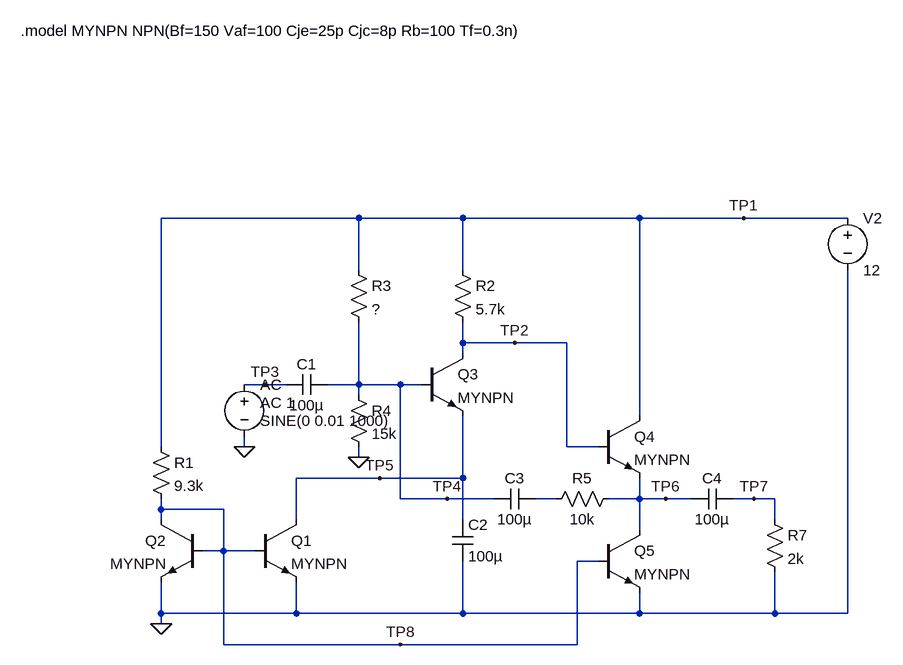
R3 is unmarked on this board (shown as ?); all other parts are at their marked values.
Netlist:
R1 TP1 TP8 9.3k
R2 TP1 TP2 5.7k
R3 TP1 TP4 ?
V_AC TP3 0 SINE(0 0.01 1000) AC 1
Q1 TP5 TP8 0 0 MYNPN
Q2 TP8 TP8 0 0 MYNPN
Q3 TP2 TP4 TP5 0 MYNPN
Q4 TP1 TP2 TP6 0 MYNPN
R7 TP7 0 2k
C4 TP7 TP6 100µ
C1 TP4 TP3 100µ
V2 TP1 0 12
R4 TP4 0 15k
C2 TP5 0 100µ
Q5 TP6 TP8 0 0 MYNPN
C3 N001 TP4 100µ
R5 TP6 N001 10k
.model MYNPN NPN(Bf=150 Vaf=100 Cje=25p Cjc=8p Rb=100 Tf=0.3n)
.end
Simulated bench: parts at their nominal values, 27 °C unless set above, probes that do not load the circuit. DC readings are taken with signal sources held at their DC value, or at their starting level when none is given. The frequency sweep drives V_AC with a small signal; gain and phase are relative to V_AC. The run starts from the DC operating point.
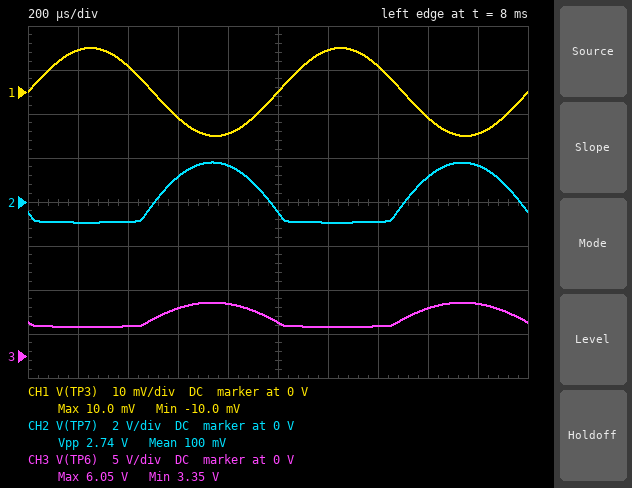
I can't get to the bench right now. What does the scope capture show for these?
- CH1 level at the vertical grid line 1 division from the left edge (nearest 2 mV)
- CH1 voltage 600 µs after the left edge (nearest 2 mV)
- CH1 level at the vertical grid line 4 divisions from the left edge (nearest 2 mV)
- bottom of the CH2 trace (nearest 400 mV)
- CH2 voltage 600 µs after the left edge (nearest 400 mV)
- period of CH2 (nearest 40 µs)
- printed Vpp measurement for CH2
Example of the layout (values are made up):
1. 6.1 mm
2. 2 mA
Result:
1. 10 mV
2. -6 mV
3. -10 mV
4. -800 mV
5. 1.2 V
6. 1.00 ms
7. 2.74 V
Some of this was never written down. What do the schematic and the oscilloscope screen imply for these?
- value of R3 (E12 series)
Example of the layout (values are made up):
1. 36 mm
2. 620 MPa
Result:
1. 22 kΩ
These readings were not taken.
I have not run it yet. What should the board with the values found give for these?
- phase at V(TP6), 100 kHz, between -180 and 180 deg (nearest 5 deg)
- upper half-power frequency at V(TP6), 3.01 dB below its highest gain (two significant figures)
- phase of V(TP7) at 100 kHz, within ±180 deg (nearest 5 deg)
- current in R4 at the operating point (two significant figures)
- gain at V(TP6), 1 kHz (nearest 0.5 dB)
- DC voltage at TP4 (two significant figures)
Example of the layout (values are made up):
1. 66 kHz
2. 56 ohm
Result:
1. 170 deg
2. 670 kHz
3. 170 deg
4. 320 µA
5. 47.5 dB
6. 4.8 V
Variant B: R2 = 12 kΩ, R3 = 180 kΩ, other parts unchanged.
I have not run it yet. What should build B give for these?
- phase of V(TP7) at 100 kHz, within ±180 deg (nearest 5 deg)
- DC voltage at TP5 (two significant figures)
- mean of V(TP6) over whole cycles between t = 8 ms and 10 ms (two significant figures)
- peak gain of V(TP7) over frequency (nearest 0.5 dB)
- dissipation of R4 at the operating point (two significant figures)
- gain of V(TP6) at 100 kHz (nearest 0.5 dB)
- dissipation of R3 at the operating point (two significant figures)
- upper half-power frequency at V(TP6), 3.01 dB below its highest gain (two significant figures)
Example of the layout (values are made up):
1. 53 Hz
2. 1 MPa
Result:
1. 170 deg
2. 77 mV
3. 1.4 V
4. 50.5 dB
5. 48 µW
6. 50.0 dB
7. 690 µW
8. 510 kHz
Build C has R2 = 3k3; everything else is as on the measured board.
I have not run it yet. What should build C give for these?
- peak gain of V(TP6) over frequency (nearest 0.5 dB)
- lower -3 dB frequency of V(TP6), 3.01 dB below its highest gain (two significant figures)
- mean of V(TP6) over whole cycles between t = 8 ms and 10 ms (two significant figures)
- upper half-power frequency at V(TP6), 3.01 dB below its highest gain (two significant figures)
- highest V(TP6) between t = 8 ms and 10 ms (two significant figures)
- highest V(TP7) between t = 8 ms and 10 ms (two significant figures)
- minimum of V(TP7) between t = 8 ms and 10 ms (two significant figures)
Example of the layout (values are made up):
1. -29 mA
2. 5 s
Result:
1. 43.0 dB
2. 93 Hz
3. 7.2 V
4. 1.6 MHz
5. 8.5 V
6. 1.3 V
7. -1.5 V
